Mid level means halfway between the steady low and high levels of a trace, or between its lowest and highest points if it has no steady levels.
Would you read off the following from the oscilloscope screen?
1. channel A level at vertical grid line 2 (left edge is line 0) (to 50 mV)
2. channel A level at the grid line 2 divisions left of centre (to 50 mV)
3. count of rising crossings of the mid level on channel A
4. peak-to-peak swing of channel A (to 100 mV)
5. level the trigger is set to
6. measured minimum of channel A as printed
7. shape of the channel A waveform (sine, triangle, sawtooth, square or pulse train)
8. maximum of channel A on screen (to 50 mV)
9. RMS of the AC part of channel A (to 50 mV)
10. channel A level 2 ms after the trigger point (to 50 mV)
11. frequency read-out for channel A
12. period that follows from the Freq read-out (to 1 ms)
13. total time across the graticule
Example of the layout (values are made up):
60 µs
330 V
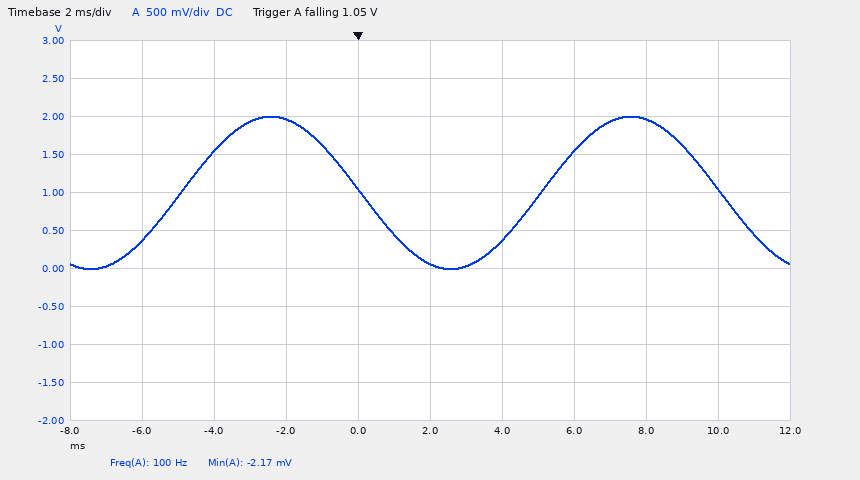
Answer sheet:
1.55 V
1.95 V
2
2.00 V
1.05 V
-2.17 mV
sine
2.00 V
700 mV
50 mV
100 Hz
10 ms
20 ms
